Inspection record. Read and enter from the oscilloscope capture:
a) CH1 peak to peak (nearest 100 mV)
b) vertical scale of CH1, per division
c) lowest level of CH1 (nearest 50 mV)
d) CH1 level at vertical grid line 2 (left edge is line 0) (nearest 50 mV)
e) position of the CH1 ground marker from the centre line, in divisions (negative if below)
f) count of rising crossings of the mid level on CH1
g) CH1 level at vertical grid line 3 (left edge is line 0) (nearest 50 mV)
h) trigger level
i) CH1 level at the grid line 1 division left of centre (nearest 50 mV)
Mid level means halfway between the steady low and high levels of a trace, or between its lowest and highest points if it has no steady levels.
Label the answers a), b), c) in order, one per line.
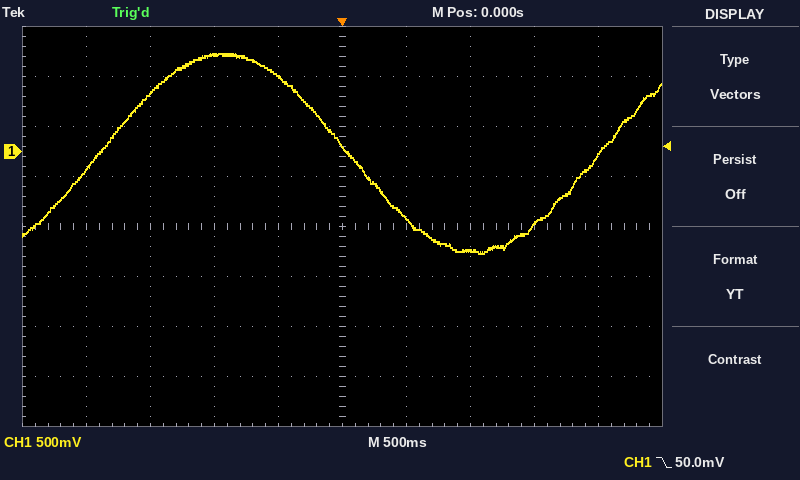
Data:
a) 2.00 V
b) 500 mV
c) -1.00 V
d) 600 mV
e) +1.5 div
f) 2
g) 950 mV
h) 50.0 mV
i) 750 mV
